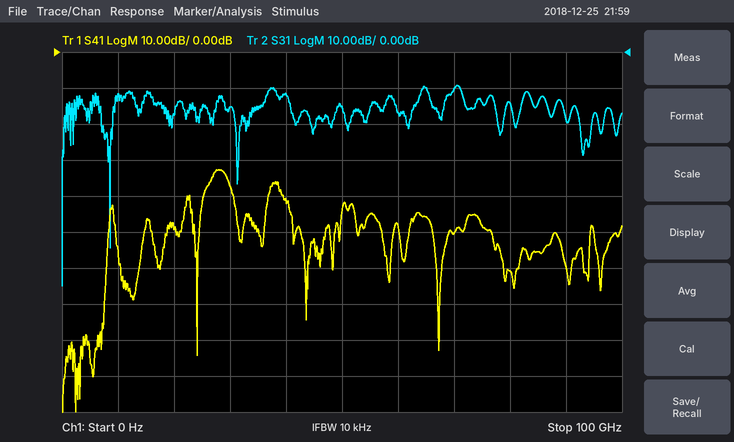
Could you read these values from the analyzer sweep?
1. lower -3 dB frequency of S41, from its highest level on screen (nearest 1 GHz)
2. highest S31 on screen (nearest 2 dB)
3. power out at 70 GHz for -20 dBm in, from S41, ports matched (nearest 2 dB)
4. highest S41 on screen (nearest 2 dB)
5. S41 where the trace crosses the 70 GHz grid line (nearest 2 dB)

27 GHz
-10 dB
-70 dBm
-32 dB
-50 dB
